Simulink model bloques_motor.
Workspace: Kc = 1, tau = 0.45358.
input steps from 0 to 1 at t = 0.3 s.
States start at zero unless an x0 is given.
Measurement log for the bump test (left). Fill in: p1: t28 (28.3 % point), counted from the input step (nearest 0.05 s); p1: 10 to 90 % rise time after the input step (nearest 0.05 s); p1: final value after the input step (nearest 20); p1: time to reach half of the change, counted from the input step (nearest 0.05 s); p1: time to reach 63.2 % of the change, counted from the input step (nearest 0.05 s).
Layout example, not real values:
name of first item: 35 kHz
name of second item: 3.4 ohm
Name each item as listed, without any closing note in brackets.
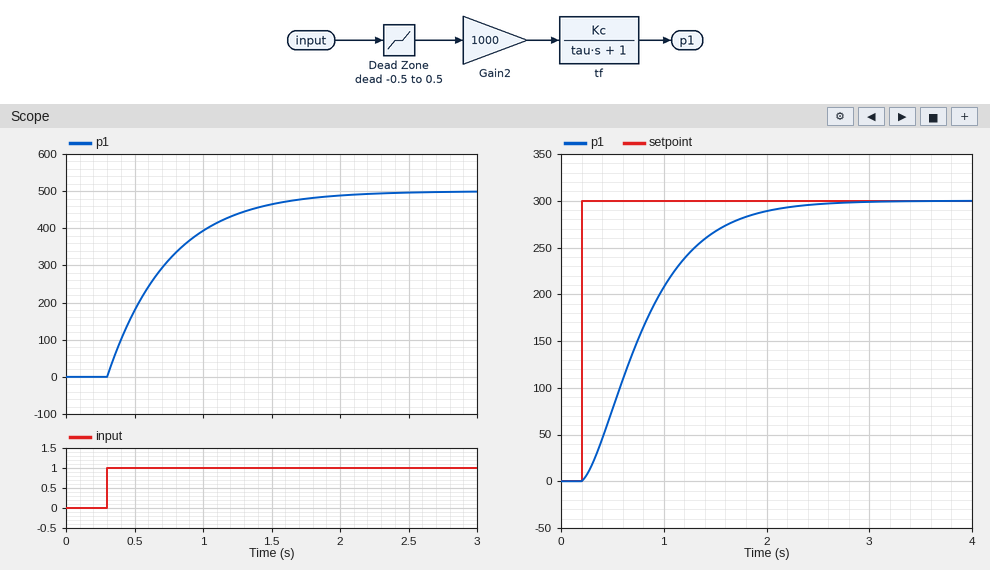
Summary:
p1: t28 (28.3 % point), counted from the input step: 0.15 s
p1: 10 to 90 % rise time after the input step: 1.00 s
p1: final value after the input step: 500
p1: time to reach half of the change, counted from the input step: 0.30 s
p1: time to reach 63.2 % of the change, counted from the input step: 0.45 s
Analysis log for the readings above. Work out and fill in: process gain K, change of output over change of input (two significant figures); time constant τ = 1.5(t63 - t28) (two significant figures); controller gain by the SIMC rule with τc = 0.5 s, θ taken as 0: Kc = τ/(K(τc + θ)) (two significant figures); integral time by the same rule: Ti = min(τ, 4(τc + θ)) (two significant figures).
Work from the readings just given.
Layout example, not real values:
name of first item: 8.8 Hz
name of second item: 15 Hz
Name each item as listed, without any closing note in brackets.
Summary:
process gain K, change of output over change of input: 500
time constant τ = 1.5(t63 - t28): 0.45 s
controller gain by the SIMC rule with τc = 0.5 s, θ taken as 0: Kc = τ/(K(τc + θ)): 0.0018
integral time by the same rule: Ti = min(τ, 4(τc + θ)): 0.45 s
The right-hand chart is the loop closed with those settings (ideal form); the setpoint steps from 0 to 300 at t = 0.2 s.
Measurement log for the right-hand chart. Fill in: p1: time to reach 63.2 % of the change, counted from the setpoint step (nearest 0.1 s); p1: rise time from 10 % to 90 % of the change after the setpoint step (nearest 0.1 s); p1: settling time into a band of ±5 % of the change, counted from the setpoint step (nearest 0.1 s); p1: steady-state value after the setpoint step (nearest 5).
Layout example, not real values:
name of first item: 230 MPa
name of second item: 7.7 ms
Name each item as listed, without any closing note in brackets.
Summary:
p1: time to reach 63.2 % of the change, counted from the setpoint step: 0.7 s
p1: rise time from 10 % to 90 % of the change after the setpoint step: 1.2 s
p1: settling time into a band of ±5 % of the change, counted from the setpoint step: 1.7 s
p1: steady-state value after the setpoint step: 300
